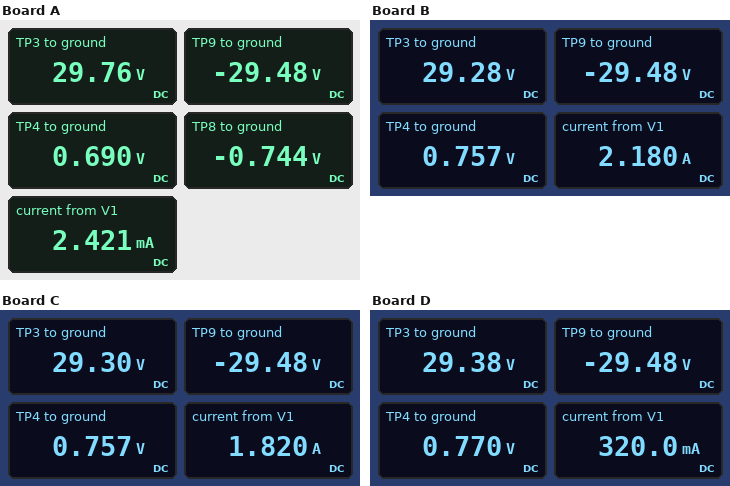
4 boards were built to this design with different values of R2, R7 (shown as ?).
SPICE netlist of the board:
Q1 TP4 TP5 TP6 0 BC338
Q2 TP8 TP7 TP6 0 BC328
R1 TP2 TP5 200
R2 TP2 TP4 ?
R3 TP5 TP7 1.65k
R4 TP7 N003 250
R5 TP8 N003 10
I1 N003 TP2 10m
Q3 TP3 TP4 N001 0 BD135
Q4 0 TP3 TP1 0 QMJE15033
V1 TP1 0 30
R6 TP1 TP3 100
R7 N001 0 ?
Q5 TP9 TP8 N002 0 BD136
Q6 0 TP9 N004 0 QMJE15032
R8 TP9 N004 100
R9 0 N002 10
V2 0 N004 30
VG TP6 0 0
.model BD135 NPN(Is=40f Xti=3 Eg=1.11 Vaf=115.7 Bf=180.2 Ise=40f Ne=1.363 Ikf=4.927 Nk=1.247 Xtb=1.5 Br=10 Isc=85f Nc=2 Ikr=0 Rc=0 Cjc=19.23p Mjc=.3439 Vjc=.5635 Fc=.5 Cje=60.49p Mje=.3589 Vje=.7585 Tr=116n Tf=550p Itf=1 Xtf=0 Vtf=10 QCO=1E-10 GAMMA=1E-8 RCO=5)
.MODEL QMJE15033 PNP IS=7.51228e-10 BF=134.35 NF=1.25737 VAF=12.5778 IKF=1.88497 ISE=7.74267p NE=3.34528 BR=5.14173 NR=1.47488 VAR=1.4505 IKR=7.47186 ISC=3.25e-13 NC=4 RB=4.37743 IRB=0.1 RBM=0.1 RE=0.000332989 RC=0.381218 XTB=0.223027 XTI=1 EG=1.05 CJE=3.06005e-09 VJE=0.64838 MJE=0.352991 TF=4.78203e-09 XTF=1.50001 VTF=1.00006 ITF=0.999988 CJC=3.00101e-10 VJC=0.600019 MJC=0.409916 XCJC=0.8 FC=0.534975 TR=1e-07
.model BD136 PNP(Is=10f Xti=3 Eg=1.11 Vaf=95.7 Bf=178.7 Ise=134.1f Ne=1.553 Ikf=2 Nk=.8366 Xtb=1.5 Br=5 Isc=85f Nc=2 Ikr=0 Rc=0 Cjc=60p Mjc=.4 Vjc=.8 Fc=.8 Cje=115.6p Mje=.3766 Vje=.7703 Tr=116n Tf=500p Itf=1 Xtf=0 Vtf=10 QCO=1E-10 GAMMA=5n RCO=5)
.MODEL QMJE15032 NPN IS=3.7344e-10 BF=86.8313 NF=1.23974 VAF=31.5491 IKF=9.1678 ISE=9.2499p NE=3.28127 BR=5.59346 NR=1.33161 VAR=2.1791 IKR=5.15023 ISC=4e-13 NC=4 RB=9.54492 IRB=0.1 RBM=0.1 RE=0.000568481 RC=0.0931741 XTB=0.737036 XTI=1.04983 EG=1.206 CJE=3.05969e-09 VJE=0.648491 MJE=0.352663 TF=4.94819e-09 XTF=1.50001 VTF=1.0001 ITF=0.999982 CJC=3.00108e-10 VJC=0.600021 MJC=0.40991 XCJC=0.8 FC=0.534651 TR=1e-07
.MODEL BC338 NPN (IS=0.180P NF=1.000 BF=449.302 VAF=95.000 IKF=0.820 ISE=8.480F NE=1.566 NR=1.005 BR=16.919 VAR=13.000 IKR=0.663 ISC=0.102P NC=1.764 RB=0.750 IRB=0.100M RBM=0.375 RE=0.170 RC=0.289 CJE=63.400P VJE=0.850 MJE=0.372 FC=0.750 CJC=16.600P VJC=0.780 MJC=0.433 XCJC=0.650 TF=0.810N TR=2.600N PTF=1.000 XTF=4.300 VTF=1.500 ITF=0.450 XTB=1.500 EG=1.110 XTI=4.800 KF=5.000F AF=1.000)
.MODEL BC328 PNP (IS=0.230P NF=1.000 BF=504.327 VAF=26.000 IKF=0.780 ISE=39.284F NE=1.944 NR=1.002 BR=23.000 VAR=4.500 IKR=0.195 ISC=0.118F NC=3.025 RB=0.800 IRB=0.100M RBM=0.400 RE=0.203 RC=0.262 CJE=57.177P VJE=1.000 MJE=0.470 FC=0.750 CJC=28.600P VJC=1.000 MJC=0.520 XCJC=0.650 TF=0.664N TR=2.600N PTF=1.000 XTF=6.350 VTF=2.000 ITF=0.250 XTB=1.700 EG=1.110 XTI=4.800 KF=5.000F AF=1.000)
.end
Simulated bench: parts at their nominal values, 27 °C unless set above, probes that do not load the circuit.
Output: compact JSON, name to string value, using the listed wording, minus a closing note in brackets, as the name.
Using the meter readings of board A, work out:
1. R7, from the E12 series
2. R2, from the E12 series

{"R7, from the E12 series": "22 Ω", "R2, from the E12 series": "12 Ω"}
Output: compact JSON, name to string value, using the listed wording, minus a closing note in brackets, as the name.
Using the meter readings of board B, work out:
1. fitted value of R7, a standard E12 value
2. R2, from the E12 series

{"fitted value of R7, a standard E12 value": "4.7 Ω", "R2, from the E12 series": "4.7 Ω"}
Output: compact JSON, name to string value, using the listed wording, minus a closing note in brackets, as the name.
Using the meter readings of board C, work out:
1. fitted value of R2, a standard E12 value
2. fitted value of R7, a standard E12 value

{"fitted value of R2, a standard E12 value": "4.7 Ω", "fitted value of R7, a standard E12 value": "5.6 Ω"}
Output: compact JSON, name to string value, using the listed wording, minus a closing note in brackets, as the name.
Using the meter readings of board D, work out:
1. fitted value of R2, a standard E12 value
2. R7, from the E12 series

{"fitted value of R2, a standard E12 value": "3.3 Ω", "R7, from the E12 series": "15 Ω"}
